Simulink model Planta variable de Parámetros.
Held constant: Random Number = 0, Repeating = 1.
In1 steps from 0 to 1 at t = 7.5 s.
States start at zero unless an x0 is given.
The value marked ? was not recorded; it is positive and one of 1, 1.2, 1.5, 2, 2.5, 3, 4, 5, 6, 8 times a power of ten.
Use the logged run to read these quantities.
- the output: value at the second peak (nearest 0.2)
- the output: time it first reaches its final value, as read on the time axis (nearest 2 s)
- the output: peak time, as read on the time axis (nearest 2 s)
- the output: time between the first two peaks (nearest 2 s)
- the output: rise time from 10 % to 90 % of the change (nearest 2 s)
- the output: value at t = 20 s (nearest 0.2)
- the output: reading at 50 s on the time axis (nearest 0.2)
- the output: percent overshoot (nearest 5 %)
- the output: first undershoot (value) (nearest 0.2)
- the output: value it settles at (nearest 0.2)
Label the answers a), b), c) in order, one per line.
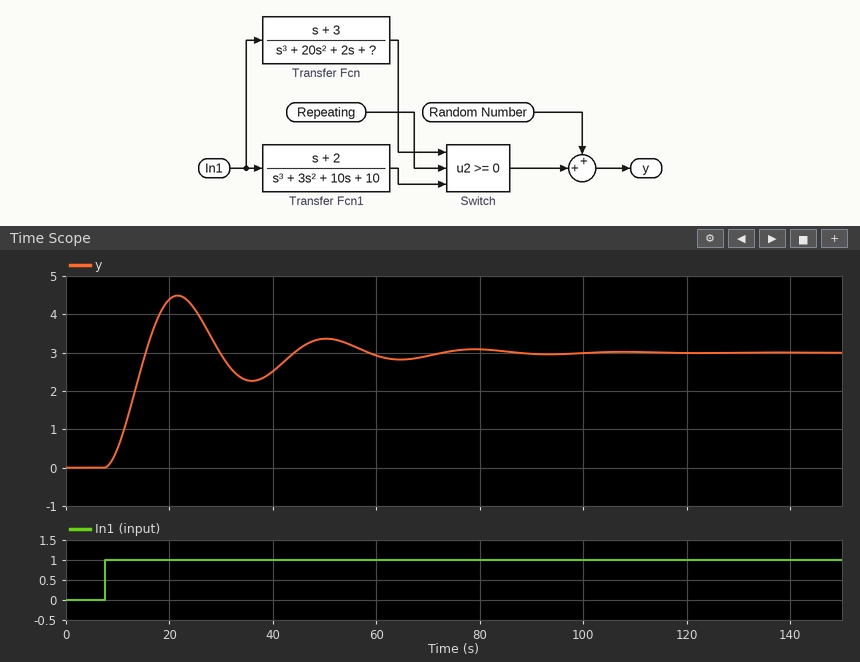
a) 3.4
b) 16 s
c) 22 s
d) 28 s
e) 6 s
f) 4.4
g) 3.4
h) 50 %
i) 2.2
j) 3.0
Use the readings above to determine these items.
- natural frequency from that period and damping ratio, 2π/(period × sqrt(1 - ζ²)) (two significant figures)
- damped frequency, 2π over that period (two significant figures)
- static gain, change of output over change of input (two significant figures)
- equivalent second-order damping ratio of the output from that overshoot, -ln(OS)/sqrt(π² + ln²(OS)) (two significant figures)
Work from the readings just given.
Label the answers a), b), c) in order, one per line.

a) 0.23 rad/s
b) 0.22 rad/s
c) 3.0
d) 0.22
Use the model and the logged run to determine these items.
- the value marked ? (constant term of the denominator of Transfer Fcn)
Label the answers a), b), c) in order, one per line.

a) 1
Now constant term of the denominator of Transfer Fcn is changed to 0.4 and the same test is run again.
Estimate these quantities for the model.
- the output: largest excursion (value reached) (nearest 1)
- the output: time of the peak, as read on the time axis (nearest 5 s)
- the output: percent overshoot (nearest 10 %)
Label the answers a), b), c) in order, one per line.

a) 10
b) 30 s
c) 30 %
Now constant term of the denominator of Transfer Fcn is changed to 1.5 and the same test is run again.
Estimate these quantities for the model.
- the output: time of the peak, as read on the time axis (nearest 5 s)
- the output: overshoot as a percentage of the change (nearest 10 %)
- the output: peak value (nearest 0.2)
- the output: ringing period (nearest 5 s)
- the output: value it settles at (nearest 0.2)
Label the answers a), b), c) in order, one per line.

a) 20 s
b) 60 %
c) 3.2
d) 25 s
e) 2.0
